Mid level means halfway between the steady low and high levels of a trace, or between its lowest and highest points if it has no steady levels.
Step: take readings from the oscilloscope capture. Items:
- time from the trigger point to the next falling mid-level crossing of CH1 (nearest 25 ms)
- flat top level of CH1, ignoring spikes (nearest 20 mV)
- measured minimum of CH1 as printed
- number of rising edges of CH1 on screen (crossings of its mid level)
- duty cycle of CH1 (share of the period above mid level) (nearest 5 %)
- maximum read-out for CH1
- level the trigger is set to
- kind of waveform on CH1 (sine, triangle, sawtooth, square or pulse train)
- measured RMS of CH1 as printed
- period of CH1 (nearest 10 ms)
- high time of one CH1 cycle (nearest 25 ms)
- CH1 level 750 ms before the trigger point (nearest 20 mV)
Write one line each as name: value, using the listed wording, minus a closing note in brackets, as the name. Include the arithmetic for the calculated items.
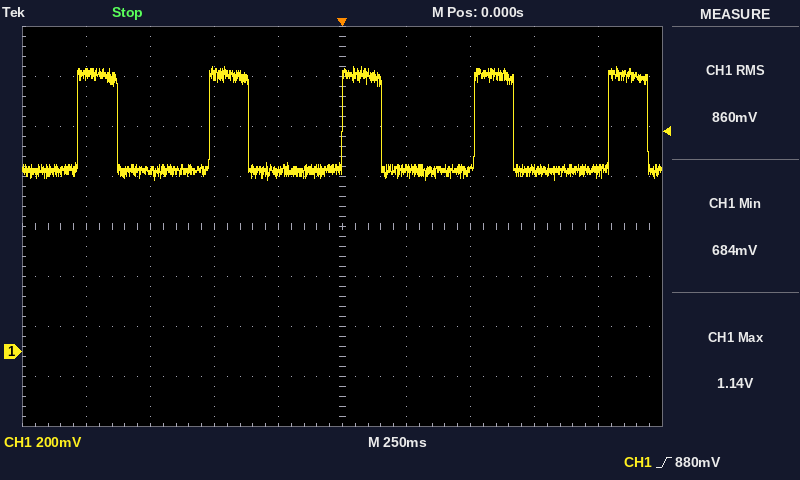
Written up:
time from the trigger point to the next falling mid-level crossing of CH1: 150 ms
flat top level of CH1, ignoring spikes: 1.10 V
measured minimum of CH1 as printed: 684 mV
number of rising edges of CH1 on screen: 5
duty cycle of CH1 (share of the period above mid level): 150 ms / 520 ms ≈ 28.8 %, so 30 % to the nearest 5 %
maximum read-out for CH1: 1.14 V
level the trigger is set to: 880 mV
kind of waveform on CH1: pulse train
measured RMS of CH1 as printed: 860 mV
period of CH1: 520 ms
high time of one CH1 cycle: 150 ms
CH1 level 750 ms before the trigger point: 720 mV
